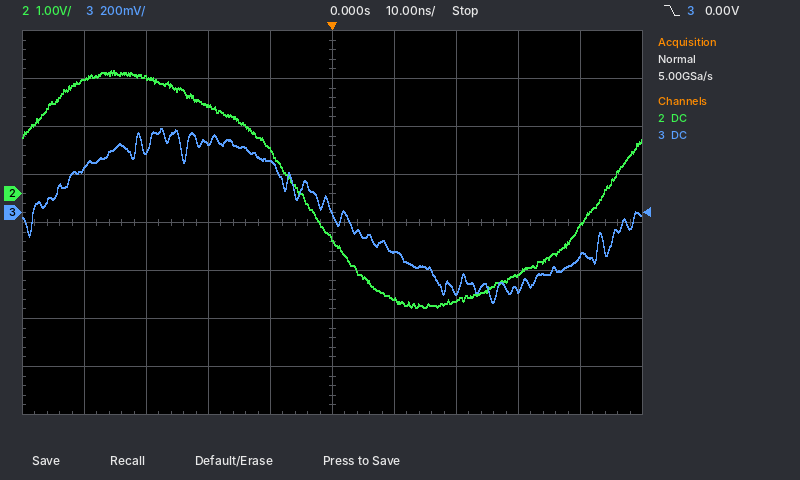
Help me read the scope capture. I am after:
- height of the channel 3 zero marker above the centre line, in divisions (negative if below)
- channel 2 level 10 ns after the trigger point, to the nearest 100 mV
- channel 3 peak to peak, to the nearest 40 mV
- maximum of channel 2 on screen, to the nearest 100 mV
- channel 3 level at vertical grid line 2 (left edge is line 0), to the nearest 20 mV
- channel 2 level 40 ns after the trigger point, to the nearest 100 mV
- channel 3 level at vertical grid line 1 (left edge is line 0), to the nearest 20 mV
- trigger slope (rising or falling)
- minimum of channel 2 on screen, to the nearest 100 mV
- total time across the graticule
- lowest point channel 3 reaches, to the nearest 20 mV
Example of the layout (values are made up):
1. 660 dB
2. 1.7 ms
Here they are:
1. +0.2 div
2. -2.2 V
3. 720 mV
4. 2.6 V
5. 260 mV
6. -700 mV
7. 180 mV
8. falling
9. -2.4 V
10. 100 ns
11. -380 mV
